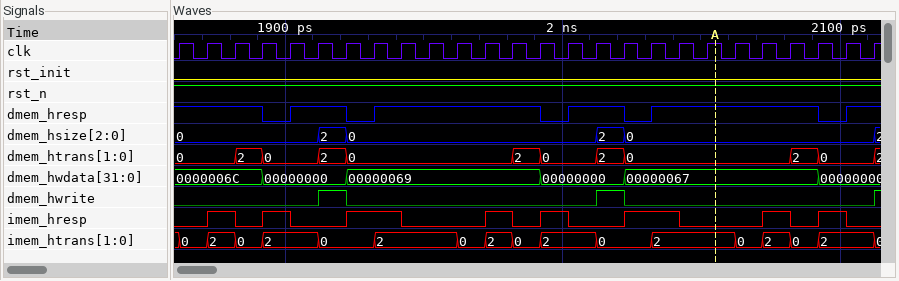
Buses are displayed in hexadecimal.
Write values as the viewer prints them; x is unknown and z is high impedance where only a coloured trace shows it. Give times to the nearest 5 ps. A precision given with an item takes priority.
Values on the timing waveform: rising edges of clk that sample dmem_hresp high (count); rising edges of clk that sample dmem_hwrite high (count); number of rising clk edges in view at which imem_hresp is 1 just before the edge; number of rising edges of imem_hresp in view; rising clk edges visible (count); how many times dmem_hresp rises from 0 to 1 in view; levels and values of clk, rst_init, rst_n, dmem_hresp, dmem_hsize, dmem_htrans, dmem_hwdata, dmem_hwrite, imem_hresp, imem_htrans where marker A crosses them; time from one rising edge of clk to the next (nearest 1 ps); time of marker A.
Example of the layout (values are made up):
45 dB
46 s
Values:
21
2
10
8
26
5
clk=1, rst_init=0, rst_n=1, dmem_hresp=1, dmem_hsize=0, dmem_htrans=0, dmem_hwdata=00000067, dmem_hwrite=0, imem_hresp=0, imem_htrans=2
10 ps
2055 ps
